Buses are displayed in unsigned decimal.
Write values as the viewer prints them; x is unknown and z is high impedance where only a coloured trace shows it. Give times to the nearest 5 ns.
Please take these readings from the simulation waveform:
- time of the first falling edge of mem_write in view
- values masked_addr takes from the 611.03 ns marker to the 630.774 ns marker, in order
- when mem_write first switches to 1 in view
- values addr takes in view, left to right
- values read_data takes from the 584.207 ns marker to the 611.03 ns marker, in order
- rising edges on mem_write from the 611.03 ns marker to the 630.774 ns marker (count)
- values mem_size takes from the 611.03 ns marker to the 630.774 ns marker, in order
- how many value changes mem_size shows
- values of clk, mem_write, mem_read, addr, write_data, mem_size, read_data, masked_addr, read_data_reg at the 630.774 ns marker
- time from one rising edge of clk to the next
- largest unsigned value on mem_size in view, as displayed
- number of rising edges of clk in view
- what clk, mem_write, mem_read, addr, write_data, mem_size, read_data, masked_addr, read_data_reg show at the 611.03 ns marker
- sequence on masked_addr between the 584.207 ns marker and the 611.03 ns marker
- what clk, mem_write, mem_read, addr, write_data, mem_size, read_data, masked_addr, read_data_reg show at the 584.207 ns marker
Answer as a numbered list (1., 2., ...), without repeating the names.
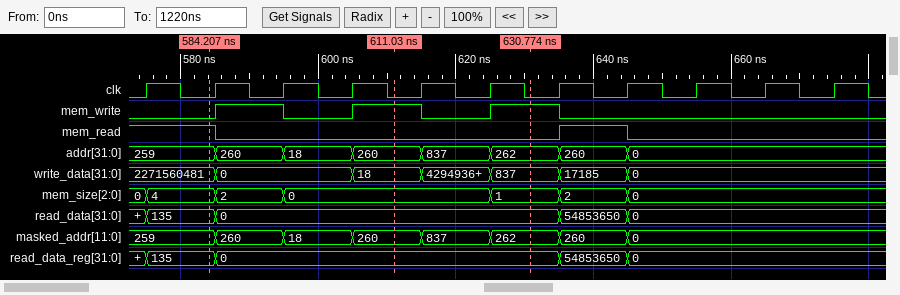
1. 595 ns
2. 260, 837, 262
3. 585 ns
4. 259, 260, 18, 260, 837, 262, 260, 0
5. 135, 0
6. 1
7. 0, 1
8. 6
9. clk=0, mem_write=1, mem_read=0, addr=262, write_data=837, mem_size=1, read_data=0, masked_addr=262, read_data_reg=0
10. 10 ns
11. 4
12. 11
13. clk=0, mem_write=1, mem_read=0, addr=260, write_data=18, mem_size=0, read_data=0, masked_addr=260, read_data_reg=0
14. 259, 260, 18, 260
15. clk=0, mem_write=0, mem_read=1, addr=259, write_data=2271560481, mem_size=4, read_data=135, masked_addr=259, read_data_reg=135
